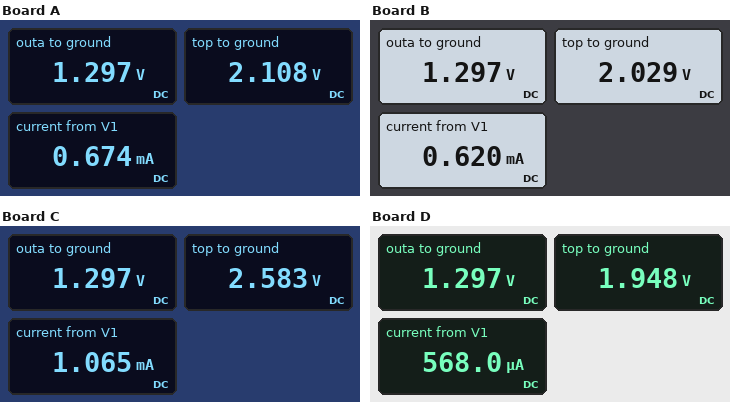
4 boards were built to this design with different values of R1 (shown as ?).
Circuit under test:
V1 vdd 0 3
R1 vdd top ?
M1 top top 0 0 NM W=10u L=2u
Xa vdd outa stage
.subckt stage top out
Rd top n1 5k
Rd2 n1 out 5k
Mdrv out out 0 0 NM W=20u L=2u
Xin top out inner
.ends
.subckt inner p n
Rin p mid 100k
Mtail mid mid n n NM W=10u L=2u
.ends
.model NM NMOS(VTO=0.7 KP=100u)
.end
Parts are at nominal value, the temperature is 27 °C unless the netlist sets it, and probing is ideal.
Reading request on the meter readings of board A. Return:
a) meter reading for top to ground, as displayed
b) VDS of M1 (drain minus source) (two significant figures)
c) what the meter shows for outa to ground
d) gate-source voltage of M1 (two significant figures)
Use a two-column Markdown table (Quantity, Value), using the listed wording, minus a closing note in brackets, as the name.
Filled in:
| Quantity | Value |
|---|---|
| meter reading for top to ground, as displayed | 2.108 V |
| VDS of M1 (drain minus source) | 2.1 V |
| what the meter shows for outa to ground | 1.297 V |
| gate-source voltage of M1 | 2.1 V |
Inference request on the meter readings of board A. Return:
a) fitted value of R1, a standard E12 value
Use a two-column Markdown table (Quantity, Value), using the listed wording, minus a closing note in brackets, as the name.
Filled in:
| Quantity | Value |
|---|---|
| fitted value of R1, a standard E12 value | 1.8 kΩ |
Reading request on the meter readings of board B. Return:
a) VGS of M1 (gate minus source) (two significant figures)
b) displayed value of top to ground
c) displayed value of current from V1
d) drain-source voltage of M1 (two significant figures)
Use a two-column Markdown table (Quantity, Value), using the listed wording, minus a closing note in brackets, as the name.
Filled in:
| Quantity | Value |
|---|---|
| VGS of M1 (gate minus source) | 2.0 V |
| displayed value of top to ground | 2.029 V |
| displayed value of current from V1 | 0.620 mA |
| drain-source voltage of M1 | 2.0 V |
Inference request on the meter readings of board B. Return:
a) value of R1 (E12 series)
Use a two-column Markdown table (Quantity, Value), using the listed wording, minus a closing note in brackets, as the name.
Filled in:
| Quantity | Value |
|---|---|
| value of R1 | 2.2 kΩ |
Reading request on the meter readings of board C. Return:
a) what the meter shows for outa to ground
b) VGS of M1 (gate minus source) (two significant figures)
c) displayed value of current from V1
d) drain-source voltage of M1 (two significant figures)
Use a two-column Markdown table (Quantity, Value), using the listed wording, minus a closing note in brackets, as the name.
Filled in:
| Quantity | Value |
|---|---|
| what the meter shows for outa to ground | 1.297 V |
| VGS of M1 (gate minus source) | 2.6 V |
| displayed value of current from V1 | 1.065 mA |
| drain-source voltage of M1 | 2.6 V |
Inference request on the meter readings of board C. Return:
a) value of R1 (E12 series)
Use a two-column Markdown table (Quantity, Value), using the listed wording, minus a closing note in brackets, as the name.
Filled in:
| Quantity | Value |
|---|---|
| value of R1 | 470 Ω |
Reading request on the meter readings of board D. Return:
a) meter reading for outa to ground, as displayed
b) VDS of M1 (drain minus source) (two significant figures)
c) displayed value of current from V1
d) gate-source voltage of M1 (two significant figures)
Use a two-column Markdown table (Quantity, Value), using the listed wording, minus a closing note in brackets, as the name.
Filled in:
| Quantity | Value |
|---|---|
| meter reading for outa to ground, as displayed | 1.297 V |
| VDS of M1 (drain minus source) | 1.9 V |
| displayed value of current from V1 | 568.0 µA |
| gate-source voltage of M1 | 1.9 V |
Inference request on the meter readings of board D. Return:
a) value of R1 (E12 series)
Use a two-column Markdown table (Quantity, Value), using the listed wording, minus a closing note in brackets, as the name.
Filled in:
| Quantity | Value |
|---|---|
| value of R1 | 2.7 kΩ |
